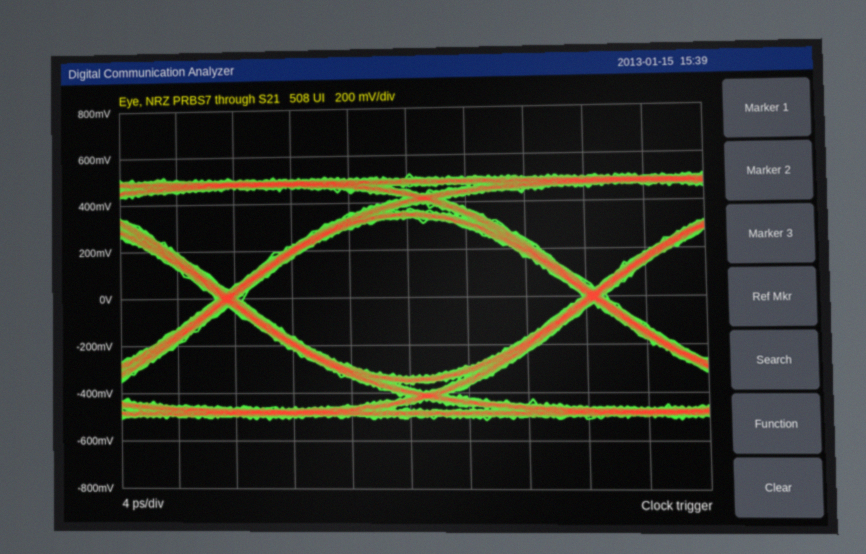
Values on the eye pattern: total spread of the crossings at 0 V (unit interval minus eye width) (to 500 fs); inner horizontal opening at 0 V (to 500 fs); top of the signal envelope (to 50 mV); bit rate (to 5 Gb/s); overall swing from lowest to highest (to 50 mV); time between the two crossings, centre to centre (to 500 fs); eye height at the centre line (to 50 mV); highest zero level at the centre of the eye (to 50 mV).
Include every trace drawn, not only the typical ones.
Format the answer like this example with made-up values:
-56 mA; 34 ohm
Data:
2.0 ps; 23.0 ps; 500 mV; 40 Gb/s; 1.05 V; 25.0 ps; 650 mV; -350 mV
